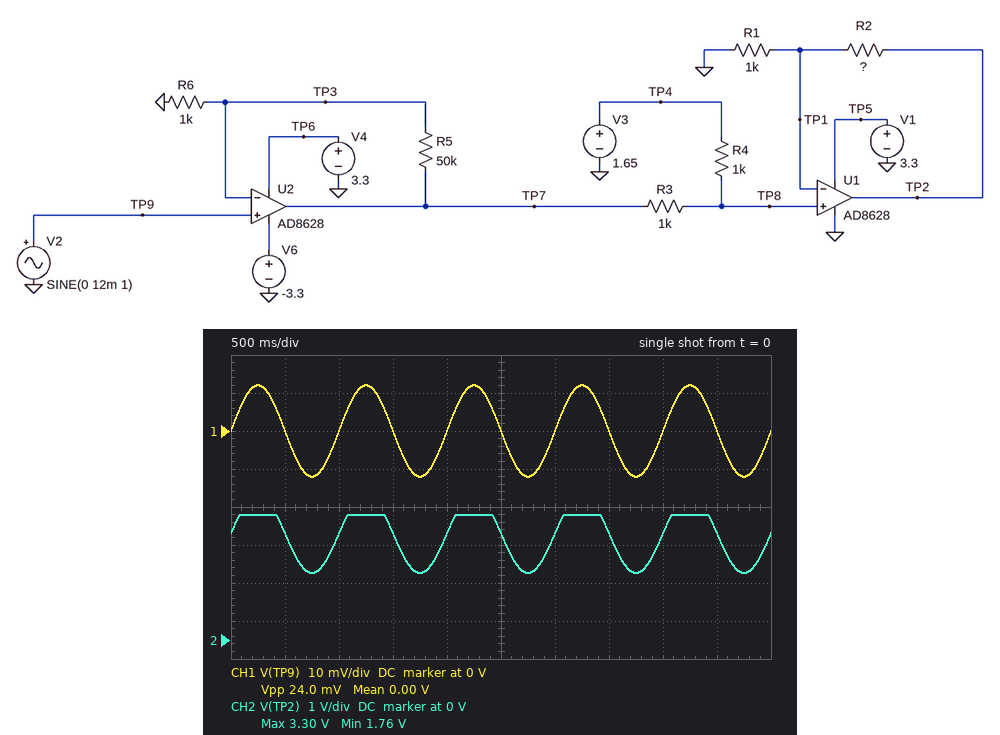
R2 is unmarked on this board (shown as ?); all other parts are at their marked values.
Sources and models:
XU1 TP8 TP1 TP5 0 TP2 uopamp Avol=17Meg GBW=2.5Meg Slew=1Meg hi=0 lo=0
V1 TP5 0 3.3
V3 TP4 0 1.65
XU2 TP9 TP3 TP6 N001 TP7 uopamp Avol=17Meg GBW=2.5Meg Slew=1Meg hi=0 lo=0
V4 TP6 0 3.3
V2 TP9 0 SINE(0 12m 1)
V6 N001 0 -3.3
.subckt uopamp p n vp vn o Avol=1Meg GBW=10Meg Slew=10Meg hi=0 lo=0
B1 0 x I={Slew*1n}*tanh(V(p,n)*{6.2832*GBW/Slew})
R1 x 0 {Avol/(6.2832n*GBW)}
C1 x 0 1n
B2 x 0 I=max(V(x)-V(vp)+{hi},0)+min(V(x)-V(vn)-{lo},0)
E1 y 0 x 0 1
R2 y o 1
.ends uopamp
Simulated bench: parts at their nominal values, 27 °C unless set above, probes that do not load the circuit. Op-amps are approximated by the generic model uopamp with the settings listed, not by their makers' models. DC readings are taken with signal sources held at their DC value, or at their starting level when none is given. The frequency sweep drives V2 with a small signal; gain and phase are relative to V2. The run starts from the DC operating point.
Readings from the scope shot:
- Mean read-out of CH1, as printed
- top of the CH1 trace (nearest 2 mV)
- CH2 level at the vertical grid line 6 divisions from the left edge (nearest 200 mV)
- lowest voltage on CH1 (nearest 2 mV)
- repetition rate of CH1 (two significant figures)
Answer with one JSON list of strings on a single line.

["0.00 V", "12 mV", "2.8 V", "-12 mV", "1.0 Hz"]
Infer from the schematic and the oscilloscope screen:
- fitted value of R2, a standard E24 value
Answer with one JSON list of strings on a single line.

["2.4 kΩ"]
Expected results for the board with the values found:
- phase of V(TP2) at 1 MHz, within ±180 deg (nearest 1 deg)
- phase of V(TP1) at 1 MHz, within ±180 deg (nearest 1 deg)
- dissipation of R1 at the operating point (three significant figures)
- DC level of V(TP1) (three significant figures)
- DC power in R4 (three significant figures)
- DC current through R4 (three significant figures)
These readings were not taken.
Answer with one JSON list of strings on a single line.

["-141 deg", "-141 deg", "681 µW", "825 mV", "681 µW", "825 µA"]
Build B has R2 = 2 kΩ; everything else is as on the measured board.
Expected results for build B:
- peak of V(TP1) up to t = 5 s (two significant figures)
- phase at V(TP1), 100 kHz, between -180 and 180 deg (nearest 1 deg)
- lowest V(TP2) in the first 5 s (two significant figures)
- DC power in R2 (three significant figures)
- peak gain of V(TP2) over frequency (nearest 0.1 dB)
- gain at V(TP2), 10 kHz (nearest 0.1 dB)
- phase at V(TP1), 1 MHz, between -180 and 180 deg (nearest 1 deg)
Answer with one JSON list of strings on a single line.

["1.1 V", "-71 deg", "1.6 V", "1.36 mW", "37.7 dB", "37.5 dB", "-137 deg"]
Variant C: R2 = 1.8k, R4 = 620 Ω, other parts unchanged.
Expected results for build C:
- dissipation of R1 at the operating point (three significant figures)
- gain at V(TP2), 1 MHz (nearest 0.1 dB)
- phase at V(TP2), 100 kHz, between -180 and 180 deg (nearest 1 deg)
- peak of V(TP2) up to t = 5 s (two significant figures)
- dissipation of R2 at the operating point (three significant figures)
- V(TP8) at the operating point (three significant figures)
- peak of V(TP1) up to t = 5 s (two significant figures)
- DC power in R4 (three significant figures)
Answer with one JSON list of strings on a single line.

["1.04 mW", "5.0 dB", "-70 deg", "3.3 V", "1.87 mW", "1.02 V", "1.2 V", "643 µW"]
